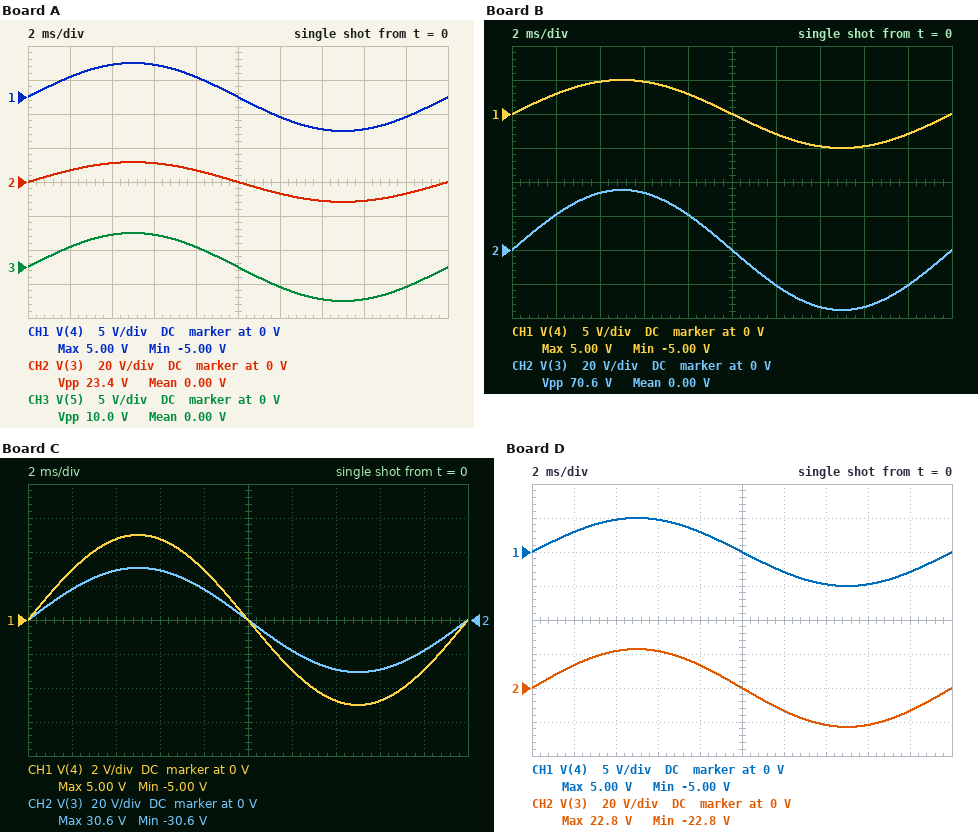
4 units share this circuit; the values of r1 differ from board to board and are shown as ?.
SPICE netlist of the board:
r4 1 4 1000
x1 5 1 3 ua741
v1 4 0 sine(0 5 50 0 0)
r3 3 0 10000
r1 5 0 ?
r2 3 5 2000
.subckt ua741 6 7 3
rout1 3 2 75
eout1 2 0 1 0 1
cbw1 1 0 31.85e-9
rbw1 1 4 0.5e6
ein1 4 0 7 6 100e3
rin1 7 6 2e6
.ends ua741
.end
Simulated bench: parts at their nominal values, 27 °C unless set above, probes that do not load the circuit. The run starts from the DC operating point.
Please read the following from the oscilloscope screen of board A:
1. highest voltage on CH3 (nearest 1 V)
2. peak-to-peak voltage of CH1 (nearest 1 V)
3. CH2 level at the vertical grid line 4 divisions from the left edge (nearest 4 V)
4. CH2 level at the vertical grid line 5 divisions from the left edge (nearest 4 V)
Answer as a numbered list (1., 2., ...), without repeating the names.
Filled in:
1. 5 V
2. 10 V
3. 8 V
4. 0 V
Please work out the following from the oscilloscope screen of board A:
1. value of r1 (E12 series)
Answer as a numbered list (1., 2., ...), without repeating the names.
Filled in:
1. 1.5 kΩ
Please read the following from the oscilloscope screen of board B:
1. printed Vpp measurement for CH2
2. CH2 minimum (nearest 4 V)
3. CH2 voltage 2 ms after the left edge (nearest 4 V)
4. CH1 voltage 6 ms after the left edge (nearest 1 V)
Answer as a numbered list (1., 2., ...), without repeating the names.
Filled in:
1. 70.6 V
2. -36 V
3. 20 V
4. 5 V
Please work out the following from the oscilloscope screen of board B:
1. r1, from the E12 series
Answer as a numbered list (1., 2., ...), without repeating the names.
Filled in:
1. 330 Ω
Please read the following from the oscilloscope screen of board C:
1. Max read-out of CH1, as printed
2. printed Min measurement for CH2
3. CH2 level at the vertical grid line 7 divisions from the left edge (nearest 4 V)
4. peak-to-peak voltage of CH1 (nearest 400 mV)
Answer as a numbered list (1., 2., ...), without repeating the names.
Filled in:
1. 5.00 V
2. -30.6 V
3. -28 V
4. 10.0 V
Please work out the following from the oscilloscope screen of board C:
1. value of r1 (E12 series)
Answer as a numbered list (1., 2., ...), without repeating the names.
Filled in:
1. 390 Ω
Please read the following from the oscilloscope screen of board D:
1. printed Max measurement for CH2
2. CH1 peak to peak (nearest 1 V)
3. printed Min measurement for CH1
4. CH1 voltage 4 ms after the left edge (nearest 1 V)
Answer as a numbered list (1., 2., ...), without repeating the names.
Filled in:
1. 22.8 V
2. 10 V
3. -5.00 V
4. 5 V
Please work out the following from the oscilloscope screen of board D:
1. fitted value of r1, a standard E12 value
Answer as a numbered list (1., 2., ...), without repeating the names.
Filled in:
1. 560 Ω
